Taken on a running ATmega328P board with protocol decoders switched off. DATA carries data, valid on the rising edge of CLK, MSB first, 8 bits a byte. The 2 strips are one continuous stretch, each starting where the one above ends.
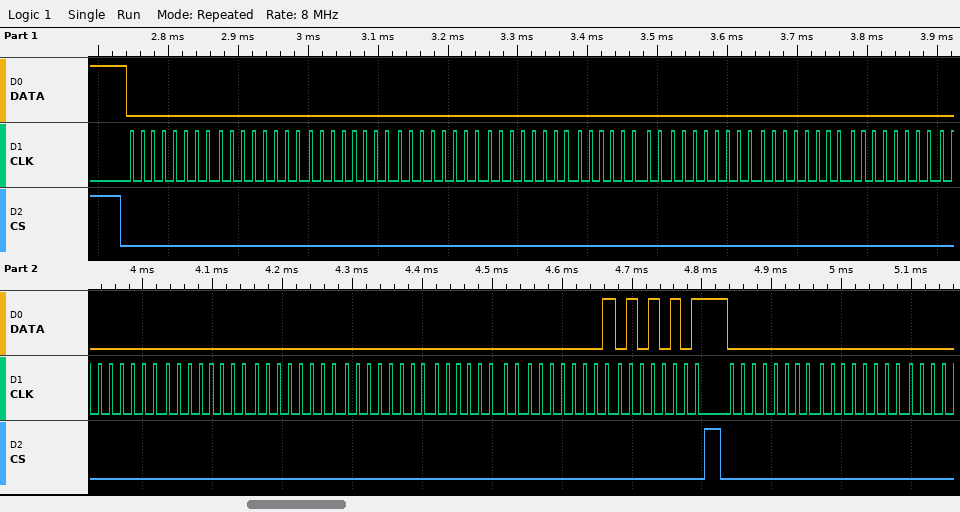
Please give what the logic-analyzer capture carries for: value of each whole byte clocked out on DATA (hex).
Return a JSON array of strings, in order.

["00 00 00 00 00 00 00 00 00 00 00 00 00 00 01 55 00 00"]
